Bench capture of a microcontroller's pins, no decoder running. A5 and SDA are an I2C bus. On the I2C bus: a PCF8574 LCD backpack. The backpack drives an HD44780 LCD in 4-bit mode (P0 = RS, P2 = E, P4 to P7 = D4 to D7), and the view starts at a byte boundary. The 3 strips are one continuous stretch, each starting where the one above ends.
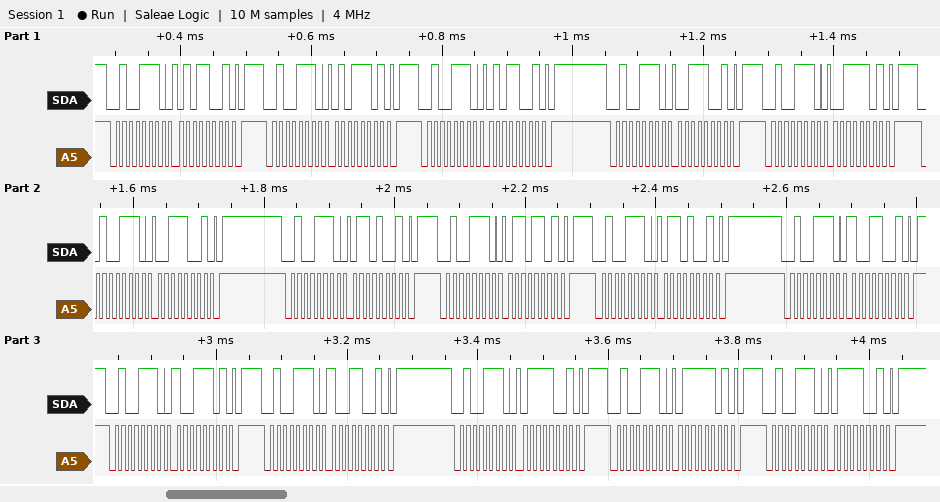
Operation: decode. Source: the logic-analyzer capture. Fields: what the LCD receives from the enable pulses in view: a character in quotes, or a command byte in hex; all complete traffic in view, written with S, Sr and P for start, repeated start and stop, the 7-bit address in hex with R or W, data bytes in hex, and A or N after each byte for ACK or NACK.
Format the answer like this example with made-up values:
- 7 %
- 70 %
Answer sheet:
- 'S' 'i'
- S 27W A 59 A P S 27W A 5D A P S 27W A 59 A P S 27W A 39 A P S 27W A 3D A P S 27W A 39 A P S 27W A 69 A P S 27W A 6D A P S 27W A 69 A P S 27W A 99 A P S 27W A 9D A P S 27W A 99 A P S 27W A 79 A P S 27W A 7D A P S 27W A 79 A P
